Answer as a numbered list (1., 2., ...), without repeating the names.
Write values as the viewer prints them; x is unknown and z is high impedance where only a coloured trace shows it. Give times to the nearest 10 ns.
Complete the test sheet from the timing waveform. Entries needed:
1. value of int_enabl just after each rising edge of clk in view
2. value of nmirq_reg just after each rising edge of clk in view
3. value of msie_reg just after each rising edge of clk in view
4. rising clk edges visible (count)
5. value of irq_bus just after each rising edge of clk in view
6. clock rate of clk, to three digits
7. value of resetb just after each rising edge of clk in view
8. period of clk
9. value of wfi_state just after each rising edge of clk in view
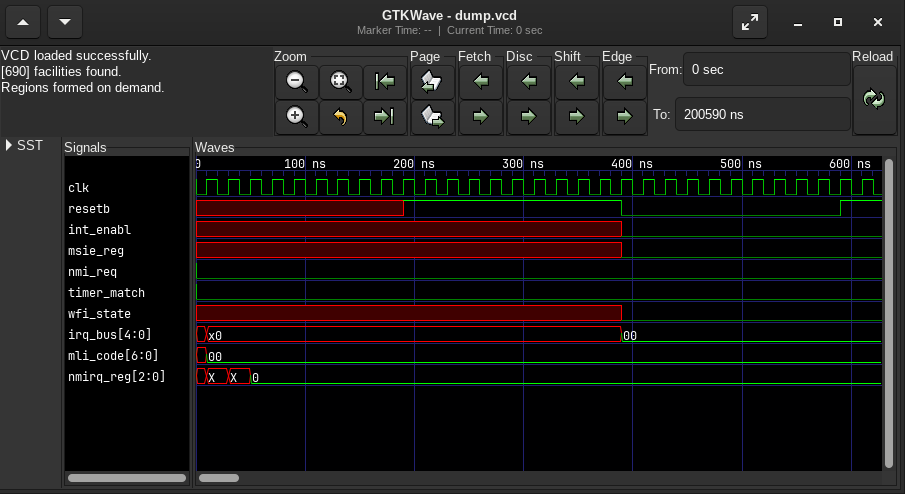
1. x x x x x x x x x x x x x x x x x x x 0 0 0 0 0 0 0 0 0 0 0 0
2. X, X, 0, 0, 0, 0, 0, 0, 0, 0, 0, 0, 0, 0, 0, 0, 0, 0, 0, 0, 0, 0, 0, 0, 0, 0, 0, 0, 0, 0, 0
3. x x x x x x x x x x x x x x x x x x x 0 0 0 0 0 0 0 0 0 0 0 0
4. 31
5. x0, x0, x0, x0, x0, x0, x0, x0, x0, x0, x0, x0, x0, x0, x0, x0, x0, x0, x0, 00, 00, 00, 00, 00, 00, 00, 00, 00, 00, 00, 00
6. 50.0 MHz
7. x x x x x x x x x 1 1 1 1 1 1 1 1 1 1 0 0 0 0 0 0 0 0 0 0 1 1
8. 20 ns
9. x x x x x x x x x x x x x x x x x x x 0 0 0 0 0 0 0 0 0 0 0 0
